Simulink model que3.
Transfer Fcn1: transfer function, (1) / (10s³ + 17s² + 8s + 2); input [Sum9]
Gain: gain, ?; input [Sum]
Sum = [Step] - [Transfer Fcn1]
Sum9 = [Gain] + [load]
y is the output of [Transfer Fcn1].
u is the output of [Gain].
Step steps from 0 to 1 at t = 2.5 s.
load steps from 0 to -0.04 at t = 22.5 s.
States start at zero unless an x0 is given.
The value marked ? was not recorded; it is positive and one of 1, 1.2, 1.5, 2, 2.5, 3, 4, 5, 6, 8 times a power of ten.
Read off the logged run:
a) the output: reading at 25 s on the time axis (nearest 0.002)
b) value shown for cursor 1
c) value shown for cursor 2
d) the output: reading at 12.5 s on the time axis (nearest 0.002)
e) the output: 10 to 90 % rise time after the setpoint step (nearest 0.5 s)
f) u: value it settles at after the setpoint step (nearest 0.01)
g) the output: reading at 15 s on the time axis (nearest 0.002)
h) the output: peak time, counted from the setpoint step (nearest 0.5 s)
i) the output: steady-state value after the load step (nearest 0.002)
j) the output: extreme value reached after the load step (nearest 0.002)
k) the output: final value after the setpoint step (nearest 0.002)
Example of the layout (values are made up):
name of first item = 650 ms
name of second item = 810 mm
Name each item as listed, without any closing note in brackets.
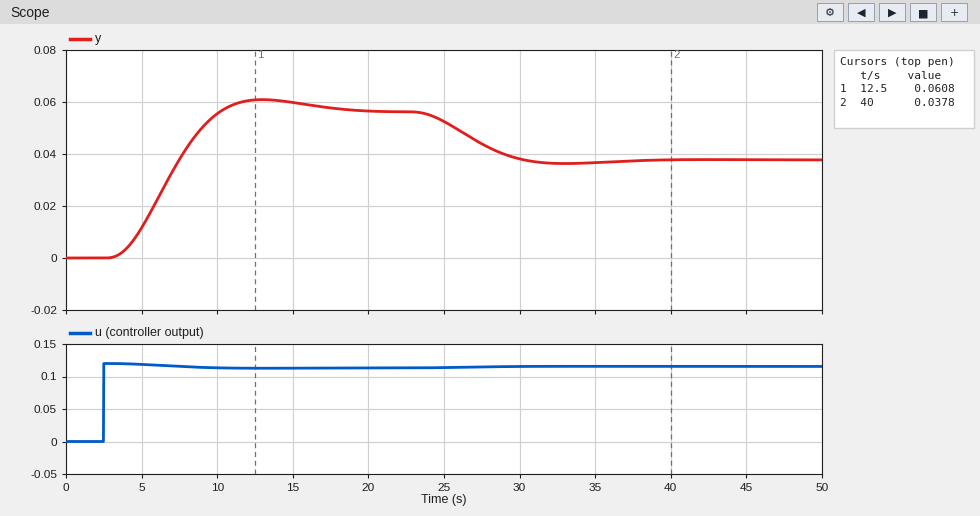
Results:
the output: reading at 25 s on the time axis = 0.052
value shown for cursor 1 = 0.0608
value shown for cursor 2 = 0.0378
the output: reading at 12.5 s on the time axis = 0.060
the output: 10 to 90 % rise time after the setpoint step = 5.0 s
u: value it settles at after the setpoint step = 0.11
the output: reading at 15 s on the time axis = 0.060
the output: peak time, counted from the setpoint step = 10.5 s
the output: steady-state value after the load step = 0.038
the output: extreme value reached after the load step = 0.036
the output: final value after the setpoint step = 0.056
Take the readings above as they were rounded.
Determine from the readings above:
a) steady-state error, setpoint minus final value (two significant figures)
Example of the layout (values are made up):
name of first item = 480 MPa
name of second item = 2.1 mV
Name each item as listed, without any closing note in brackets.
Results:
steady-state error, setpoint minus final value = 0.94
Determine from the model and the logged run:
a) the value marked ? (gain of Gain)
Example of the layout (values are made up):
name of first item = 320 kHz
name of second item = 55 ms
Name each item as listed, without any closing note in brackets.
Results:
the value marked ? = 0.12
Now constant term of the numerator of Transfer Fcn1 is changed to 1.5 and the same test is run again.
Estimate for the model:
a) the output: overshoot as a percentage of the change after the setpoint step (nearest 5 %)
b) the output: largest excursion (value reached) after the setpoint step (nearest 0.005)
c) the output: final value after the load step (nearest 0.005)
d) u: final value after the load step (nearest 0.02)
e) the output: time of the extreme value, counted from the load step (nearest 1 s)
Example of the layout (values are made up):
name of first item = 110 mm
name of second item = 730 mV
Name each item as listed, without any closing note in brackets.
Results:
the output: overshoot as a percentage of the change after the setpoint step = 10 %
the output: largest excursion (value reached) after the setpoint step = 0.090
the output: final value after the load step = 0.055
u: final value after the load step = 0.12
the output: time of the extreme value, counted from the load step = 10 s
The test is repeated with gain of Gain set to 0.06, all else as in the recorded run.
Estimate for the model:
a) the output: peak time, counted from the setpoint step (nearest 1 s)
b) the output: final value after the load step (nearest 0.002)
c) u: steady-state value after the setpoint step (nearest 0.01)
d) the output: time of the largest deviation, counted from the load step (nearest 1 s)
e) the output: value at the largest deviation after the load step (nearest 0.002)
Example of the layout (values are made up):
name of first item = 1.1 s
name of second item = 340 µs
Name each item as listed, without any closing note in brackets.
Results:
the output: peak time, counted from the setpoint step = 11 s
the output: final value after the load step = 0.010
u: steady-state value after the setpoint step = 0.06
the output: time of the largest deviation, counted from the load step = 11 s
the output: value at the largest deviation after the load step = 0.008
